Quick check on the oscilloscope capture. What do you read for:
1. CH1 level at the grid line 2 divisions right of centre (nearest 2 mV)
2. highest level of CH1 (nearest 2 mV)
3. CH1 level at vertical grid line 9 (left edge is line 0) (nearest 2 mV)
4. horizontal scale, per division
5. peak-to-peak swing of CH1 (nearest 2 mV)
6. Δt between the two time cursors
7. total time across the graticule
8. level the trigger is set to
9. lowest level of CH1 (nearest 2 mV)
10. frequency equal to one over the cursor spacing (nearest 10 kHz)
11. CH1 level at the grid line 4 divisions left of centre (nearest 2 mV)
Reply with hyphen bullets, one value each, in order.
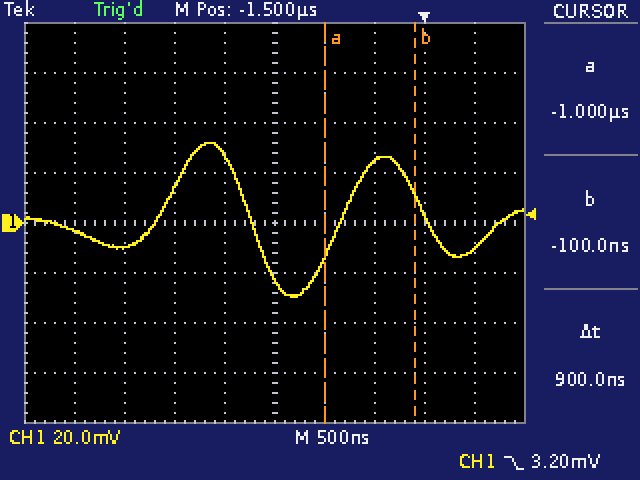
- 24 mV
- 32 mV
- -10 mV
- 500 ns
- 62 mV
- 900 ns
- 5 µs
- 3.20 mV
- -30 mV
- 1.11 MHz
- -4 mV
